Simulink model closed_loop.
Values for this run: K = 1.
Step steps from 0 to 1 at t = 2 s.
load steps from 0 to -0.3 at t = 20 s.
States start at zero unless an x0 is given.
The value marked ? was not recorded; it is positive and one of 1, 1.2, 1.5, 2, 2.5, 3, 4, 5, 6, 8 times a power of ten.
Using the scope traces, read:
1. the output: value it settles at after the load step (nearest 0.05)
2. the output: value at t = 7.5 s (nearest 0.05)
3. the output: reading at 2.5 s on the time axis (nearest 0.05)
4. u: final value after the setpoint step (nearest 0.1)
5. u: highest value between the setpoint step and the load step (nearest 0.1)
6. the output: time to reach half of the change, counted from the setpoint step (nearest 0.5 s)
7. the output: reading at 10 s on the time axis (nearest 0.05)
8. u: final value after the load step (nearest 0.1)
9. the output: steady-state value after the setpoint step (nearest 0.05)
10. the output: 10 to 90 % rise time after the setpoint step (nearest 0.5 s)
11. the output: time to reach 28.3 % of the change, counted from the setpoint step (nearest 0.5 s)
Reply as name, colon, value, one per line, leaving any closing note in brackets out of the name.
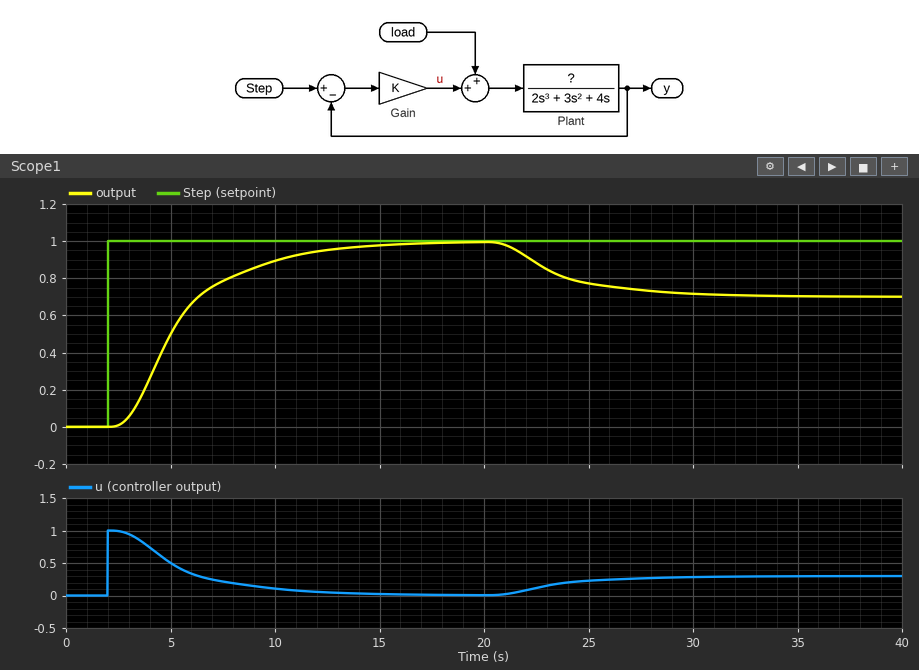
the output: value it settles at after the load step: 0.70
the output: value at t = 7.5 s: 0.80
the output: reading at 2.5 s on the time axis: 0.00
u: final value after the setpoint step: 0.0
u: highest value between the setpoint step and the load step: 1.0
the output: time to reach half of the change, counted from the setpoint step: 3.0 s
the output: reading at 10 s on the time axis: 0.90
u: final value after the load step: 0.3
the output: steady-state value after the setpoint step: 1.00
the output: 10 to 90 % rise time after the setpoint step: 7.0 s
the output: time to reach 28.3 % of the change, counted from the setpoint step: 2.0 s
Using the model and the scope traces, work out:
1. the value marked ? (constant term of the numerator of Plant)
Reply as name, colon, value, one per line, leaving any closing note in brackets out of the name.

the value marked ?: 1
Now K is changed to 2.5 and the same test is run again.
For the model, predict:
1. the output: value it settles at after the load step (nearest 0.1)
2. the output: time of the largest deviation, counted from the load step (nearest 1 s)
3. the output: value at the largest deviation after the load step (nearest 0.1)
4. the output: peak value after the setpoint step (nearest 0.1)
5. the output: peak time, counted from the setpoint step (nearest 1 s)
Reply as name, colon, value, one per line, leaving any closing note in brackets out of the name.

the output: value it settles at after the load step: 0.9
the output: time of the largest deviation, counted from the load step: 4 s
the output: value at the largest deviation after the load step: 0.9
the output: peak value after the setpoint step: 1.2
the output: peak time, counted from the setpoint step: 4 s
